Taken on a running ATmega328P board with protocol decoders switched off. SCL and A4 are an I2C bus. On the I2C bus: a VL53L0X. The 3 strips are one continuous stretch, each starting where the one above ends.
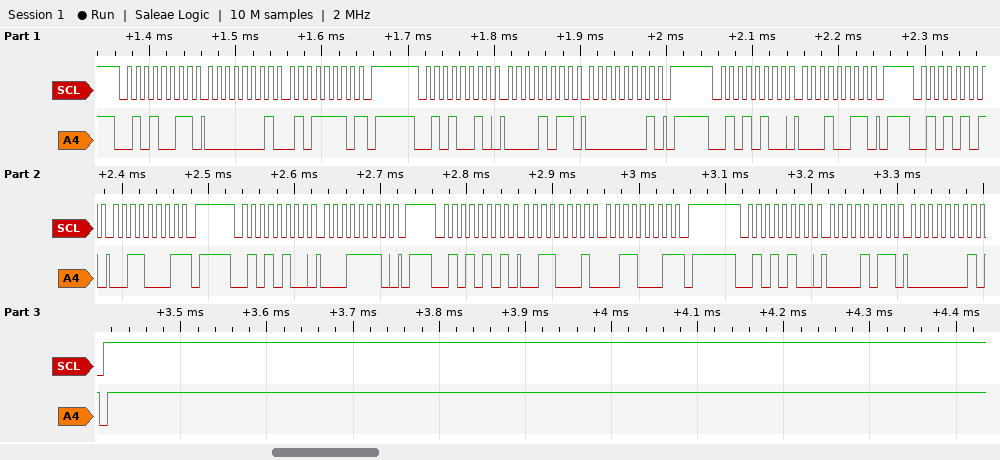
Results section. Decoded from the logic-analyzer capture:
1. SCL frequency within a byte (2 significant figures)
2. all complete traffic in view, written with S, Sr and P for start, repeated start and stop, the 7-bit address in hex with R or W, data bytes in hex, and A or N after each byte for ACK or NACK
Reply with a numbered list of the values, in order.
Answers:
1. 100 kHz
2. S 29R A 01 A 5E N P S 29W A 0B A 01 A P S 2AW A 13 A P S 2AR A 31 N P S 2AW A 1E A P S 2AR A 31 A 31 N P S 2AW A 0B A 01 A P
